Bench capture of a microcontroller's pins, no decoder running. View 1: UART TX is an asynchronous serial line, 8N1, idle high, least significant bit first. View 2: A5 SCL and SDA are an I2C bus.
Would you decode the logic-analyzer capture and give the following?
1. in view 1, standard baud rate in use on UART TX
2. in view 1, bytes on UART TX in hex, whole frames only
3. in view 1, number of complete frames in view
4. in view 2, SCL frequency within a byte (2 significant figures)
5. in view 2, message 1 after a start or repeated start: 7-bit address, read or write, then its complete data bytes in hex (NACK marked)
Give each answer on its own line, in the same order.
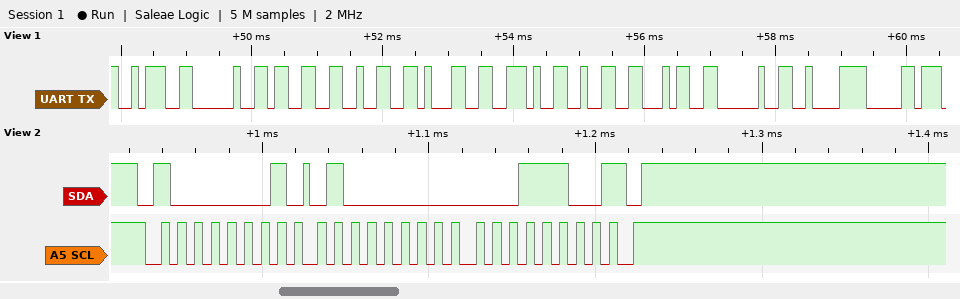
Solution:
9600 baud
3A 20 33 32 31 2E 32 34 20 C2 B0
11
100 kHz
0x40 read: 40 1C NACK
